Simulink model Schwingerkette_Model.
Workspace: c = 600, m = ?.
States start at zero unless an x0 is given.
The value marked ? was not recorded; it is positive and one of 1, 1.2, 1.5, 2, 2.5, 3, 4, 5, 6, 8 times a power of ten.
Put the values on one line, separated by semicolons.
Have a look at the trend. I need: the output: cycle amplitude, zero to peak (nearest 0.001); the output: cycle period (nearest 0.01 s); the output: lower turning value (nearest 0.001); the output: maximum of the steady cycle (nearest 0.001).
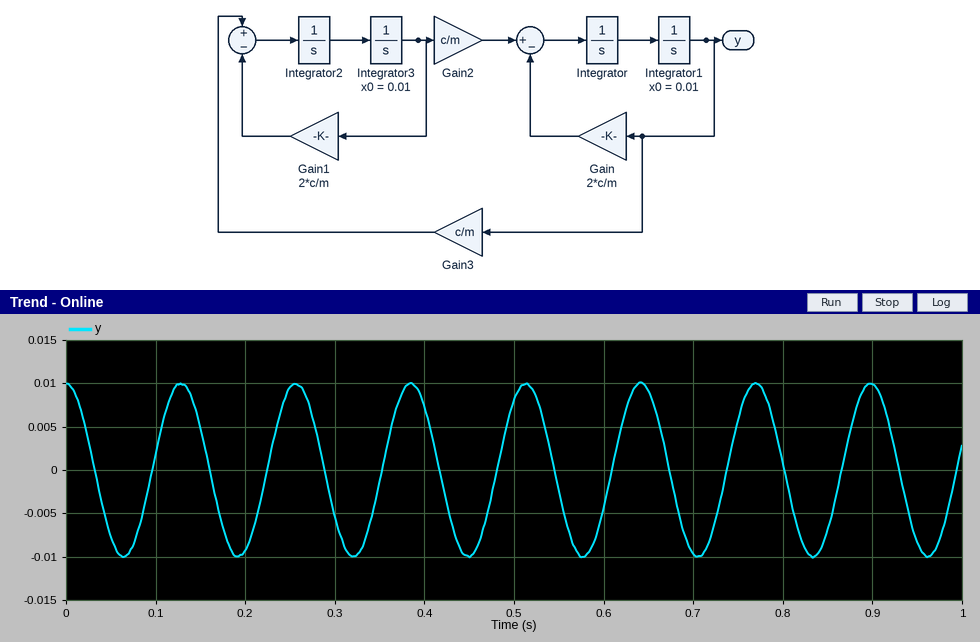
0.010; 0.13 s; -0.010; 0.010
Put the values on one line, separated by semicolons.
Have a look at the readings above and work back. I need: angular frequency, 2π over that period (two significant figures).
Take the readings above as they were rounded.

48 rad/s
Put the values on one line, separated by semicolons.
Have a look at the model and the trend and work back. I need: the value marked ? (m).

0.25
